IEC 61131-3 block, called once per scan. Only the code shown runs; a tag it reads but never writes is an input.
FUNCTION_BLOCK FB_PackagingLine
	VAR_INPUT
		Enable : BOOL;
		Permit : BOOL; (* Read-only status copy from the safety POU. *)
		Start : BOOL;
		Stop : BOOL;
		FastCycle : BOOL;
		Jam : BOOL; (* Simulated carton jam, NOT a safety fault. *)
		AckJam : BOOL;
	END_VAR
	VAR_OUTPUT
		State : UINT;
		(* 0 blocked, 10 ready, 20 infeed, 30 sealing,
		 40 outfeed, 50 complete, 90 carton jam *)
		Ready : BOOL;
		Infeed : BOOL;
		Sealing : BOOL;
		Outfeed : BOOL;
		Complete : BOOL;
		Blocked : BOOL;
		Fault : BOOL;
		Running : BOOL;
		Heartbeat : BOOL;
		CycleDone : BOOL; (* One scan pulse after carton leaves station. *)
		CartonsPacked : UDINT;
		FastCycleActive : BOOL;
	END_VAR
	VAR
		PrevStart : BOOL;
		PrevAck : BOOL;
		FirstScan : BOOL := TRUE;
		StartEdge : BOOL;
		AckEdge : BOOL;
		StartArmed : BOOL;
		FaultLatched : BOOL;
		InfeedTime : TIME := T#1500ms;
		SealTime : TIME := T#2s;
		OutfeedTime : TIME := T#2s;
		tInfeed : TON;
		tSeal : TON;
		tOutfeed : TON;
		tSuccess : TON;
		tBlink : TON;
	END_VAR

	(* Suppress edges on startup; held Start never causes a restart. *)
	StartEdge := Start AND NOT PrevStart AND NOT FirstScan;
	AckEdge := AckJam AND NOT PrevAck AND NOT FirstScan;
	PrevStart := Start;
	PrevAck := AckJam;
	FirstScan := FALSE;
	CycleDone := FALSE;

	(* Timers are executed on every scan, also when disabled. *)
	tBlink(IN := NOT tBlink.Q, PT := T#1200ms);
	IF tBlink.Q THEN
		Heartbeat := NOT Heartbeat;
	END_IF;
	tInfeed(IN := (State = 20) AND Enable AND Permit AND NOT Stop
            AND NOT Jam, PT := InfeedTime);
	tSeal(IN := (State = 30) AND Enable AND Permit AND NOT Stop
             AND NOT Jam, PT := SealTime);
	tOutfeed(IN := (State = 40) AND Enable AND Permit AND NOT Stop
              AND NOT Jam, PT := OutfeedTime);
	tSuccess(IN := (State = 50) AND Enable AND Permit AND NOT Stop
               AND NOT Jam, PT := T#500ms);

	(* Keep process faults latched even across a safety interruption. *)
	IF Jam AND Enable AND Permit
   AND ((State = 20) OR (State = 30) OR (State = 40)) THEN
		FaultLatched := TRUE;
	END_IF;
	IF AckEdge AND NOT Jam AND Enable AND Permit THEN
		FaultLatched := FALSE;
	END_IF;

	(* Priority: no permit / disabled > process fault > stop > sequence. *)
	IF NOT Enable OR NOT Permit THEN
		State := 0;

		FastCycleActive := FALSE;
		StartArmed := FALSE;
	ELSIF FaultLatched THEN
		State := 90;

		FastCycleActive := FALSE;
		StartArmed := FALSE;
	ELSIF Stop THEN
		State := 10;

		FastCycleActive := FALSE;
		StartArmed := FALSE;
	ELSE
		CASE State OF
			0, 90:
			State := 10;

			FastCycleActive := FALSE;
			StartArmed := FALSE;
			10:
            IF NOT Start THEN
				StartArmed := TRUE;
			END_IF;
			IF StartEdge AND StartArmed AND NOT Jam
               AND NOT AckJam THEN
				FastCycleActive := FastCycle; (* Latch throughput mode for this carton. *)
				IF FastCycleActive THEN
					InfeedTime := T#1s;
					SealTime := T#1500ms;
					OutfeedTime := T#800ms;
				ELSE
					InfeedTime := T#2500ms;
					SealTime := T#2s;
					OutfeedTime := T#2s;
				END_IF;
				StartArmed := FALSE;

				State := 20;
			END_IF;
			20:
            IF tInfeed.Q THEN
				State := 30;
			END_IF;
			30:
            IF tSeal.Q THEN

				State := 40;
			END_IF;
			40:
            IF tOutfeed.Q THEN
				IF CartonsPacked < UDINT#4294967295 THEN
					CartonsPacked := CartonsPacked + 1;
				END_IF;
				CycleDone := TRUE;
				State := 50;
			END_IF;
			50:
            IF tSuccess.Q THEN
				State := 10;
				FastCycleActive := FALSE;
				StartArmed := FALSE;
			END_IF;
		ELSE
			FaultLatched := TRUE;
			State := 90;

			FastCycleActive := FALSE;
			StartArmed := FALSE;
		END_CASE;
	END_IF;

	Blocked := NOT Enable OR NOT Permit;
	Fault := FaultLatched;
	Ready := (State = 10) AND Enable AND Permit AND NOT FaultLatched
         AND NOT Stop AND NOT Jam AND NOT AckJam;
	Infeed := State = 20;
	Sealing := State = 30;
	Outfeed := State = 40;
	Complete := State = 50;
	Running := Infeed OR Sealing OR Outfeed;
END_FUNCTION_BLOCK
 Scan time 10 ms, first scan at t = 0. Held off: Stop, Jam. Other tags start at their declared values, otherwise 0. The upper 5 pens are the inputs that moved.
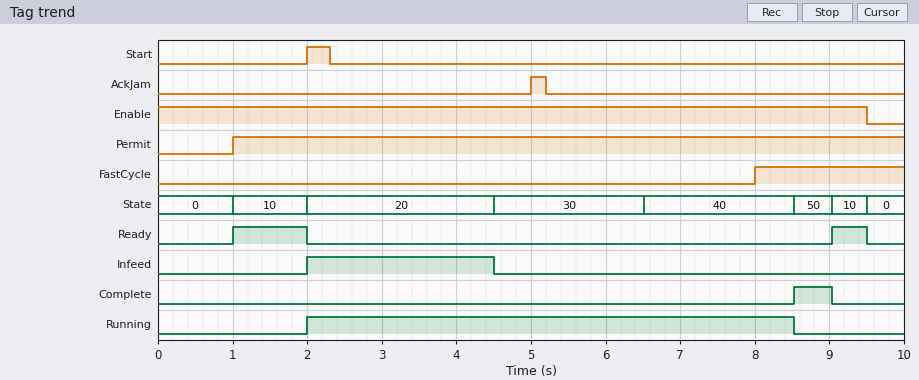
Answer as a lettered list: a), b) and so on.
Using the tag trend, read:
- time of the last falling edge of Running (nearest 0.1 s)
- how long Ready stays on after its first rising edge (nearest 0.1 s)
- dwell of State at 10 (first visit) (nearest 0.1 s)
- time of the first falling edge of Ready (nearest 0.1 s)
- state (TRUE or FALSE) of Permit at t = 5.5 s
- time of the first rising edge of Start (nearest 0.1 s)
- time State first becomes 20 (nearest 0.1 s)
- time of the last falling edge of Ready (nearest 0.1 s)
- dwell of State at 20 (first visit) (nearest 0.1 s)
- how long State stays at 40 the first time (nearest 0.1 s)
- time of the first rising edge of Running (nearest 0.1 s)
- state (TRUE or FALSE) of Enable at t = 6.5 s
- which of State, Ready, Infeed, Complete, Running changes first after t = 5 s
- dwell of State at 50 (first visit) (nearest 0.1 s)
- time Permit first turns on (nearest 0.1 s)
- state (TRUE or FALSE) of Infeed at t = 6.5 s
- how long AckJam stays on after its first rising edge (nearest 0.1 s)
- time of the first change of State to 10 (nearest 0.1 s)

a) 8.5 s
b) 1.0 s
c) 1.0 s
d) 2.0 s
e) TRUE
f) 2.0 s
g) 2.0 s
h) 9.5 s
i) 2.5 s
j) 2.0 s
k) 2.0 s
l) TRUE
m) State
n) 0.5 s
o) 1.0 s
p) FALSE
q) 0.2 s
r) 1.0 s
